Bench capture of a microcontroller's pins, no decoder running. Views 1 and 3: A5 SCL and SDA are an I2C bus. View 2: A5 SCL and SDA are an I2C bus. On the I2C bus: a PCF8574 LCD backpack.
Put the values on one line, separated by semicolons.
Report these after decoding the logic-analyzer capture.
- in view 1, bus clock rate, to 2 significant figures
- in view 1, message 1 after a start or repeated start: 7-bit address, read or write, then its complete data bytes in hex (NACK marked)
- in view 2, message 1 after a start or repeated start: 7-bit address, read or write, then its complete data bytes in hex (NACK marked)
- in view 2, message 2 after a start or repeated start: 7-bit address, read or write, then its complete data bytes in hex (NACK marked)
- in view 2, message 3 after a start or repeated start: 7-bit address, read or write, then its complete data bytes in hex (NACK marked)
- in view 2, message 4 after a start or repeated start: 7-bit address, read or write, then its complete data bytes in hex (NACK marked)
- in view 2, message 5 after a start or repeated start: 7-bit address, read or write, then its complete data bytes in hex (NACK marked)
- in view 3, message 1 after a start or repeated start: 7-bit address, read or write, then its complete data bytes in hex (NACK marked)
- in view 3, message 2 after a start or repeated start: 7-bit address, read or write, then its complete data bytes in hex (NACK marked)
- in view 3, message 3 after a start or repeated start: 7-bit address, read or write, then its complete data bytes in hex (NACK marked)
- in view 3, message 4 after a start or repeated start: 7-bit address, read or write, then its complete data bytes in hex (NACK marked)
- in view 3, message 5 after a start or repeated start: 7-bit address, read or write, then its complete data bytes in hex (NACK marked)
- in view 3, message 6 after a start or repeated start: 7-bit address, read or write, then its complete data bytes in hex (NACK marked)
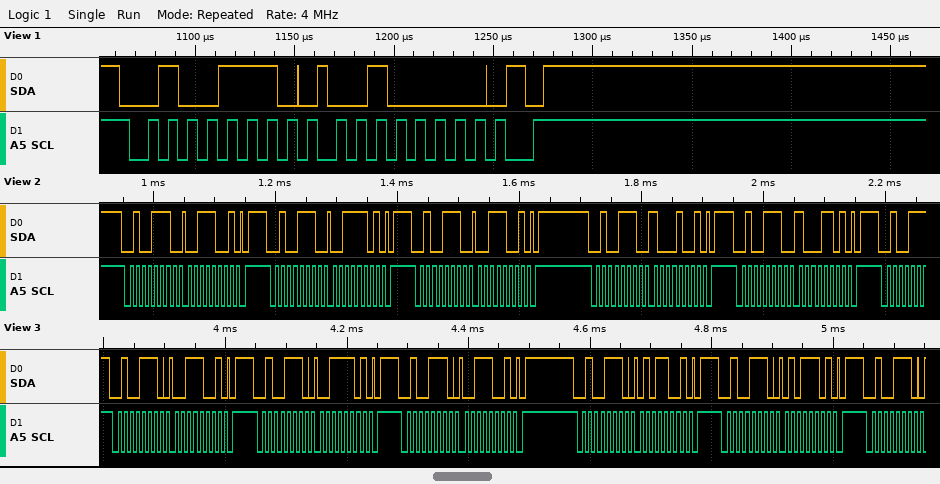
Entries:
100 kHz; 0x27 write: 20; 0x27 write: 39; 0x27 write: 3D; 0x27 write: 39; 0x27 write: 89; 0x27 write: 8D; 0x27 write: 39; 0x27 write: 3D; 0x27 write: 39; 0x27 write: 59; 0x27 write: 5D; 0x27 write
